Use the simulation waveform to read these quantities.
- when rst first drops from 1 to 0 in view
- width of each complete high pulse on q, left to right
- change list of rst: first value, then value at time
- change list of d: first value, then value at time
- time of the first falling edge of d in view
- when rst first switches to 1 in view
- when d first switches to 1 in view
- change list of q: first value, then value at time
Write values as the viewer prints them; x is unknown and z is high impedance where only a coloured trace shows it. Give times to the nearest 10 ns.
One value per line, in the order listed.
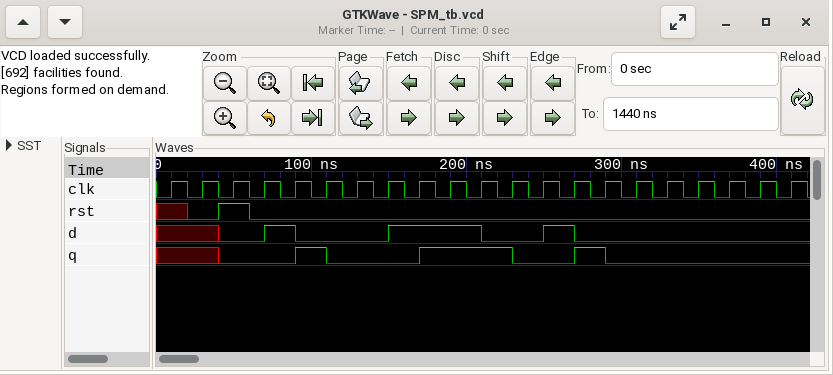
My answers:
60 ns
20 ns, 60 ns, 20 ns
x, 0 at 20 ns, 1 at 40 ns, 0 at 60 ns
x, 0 at 40 ns, 1 at 70 ns, 0 at 90 ns, 1 at 150 ns, 0 at 210 ns, 1 at 250 ns, 0 at 270 ns
90 ns
40 ns
70 ns
x, 0 at 40 ns, 1 at 90 ns, 0 at 110 ns, 1 at 170 ns, 0 at 230 ns, 1 at 270 ns, 0 at 290 ns
